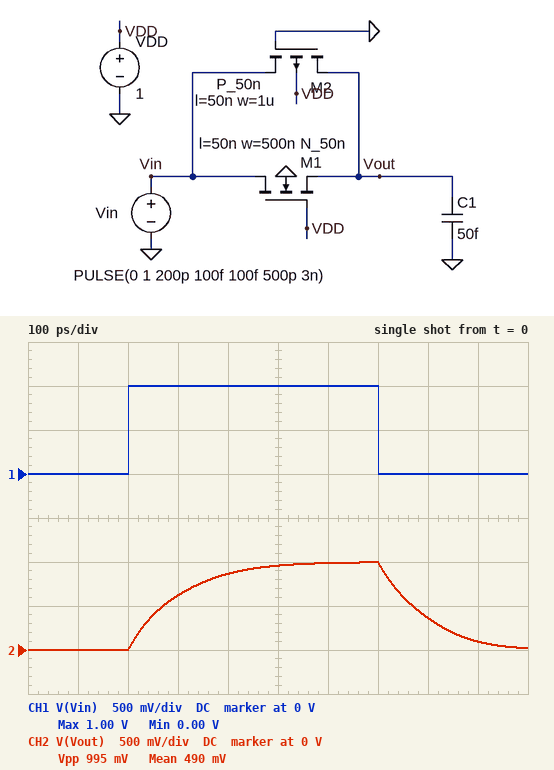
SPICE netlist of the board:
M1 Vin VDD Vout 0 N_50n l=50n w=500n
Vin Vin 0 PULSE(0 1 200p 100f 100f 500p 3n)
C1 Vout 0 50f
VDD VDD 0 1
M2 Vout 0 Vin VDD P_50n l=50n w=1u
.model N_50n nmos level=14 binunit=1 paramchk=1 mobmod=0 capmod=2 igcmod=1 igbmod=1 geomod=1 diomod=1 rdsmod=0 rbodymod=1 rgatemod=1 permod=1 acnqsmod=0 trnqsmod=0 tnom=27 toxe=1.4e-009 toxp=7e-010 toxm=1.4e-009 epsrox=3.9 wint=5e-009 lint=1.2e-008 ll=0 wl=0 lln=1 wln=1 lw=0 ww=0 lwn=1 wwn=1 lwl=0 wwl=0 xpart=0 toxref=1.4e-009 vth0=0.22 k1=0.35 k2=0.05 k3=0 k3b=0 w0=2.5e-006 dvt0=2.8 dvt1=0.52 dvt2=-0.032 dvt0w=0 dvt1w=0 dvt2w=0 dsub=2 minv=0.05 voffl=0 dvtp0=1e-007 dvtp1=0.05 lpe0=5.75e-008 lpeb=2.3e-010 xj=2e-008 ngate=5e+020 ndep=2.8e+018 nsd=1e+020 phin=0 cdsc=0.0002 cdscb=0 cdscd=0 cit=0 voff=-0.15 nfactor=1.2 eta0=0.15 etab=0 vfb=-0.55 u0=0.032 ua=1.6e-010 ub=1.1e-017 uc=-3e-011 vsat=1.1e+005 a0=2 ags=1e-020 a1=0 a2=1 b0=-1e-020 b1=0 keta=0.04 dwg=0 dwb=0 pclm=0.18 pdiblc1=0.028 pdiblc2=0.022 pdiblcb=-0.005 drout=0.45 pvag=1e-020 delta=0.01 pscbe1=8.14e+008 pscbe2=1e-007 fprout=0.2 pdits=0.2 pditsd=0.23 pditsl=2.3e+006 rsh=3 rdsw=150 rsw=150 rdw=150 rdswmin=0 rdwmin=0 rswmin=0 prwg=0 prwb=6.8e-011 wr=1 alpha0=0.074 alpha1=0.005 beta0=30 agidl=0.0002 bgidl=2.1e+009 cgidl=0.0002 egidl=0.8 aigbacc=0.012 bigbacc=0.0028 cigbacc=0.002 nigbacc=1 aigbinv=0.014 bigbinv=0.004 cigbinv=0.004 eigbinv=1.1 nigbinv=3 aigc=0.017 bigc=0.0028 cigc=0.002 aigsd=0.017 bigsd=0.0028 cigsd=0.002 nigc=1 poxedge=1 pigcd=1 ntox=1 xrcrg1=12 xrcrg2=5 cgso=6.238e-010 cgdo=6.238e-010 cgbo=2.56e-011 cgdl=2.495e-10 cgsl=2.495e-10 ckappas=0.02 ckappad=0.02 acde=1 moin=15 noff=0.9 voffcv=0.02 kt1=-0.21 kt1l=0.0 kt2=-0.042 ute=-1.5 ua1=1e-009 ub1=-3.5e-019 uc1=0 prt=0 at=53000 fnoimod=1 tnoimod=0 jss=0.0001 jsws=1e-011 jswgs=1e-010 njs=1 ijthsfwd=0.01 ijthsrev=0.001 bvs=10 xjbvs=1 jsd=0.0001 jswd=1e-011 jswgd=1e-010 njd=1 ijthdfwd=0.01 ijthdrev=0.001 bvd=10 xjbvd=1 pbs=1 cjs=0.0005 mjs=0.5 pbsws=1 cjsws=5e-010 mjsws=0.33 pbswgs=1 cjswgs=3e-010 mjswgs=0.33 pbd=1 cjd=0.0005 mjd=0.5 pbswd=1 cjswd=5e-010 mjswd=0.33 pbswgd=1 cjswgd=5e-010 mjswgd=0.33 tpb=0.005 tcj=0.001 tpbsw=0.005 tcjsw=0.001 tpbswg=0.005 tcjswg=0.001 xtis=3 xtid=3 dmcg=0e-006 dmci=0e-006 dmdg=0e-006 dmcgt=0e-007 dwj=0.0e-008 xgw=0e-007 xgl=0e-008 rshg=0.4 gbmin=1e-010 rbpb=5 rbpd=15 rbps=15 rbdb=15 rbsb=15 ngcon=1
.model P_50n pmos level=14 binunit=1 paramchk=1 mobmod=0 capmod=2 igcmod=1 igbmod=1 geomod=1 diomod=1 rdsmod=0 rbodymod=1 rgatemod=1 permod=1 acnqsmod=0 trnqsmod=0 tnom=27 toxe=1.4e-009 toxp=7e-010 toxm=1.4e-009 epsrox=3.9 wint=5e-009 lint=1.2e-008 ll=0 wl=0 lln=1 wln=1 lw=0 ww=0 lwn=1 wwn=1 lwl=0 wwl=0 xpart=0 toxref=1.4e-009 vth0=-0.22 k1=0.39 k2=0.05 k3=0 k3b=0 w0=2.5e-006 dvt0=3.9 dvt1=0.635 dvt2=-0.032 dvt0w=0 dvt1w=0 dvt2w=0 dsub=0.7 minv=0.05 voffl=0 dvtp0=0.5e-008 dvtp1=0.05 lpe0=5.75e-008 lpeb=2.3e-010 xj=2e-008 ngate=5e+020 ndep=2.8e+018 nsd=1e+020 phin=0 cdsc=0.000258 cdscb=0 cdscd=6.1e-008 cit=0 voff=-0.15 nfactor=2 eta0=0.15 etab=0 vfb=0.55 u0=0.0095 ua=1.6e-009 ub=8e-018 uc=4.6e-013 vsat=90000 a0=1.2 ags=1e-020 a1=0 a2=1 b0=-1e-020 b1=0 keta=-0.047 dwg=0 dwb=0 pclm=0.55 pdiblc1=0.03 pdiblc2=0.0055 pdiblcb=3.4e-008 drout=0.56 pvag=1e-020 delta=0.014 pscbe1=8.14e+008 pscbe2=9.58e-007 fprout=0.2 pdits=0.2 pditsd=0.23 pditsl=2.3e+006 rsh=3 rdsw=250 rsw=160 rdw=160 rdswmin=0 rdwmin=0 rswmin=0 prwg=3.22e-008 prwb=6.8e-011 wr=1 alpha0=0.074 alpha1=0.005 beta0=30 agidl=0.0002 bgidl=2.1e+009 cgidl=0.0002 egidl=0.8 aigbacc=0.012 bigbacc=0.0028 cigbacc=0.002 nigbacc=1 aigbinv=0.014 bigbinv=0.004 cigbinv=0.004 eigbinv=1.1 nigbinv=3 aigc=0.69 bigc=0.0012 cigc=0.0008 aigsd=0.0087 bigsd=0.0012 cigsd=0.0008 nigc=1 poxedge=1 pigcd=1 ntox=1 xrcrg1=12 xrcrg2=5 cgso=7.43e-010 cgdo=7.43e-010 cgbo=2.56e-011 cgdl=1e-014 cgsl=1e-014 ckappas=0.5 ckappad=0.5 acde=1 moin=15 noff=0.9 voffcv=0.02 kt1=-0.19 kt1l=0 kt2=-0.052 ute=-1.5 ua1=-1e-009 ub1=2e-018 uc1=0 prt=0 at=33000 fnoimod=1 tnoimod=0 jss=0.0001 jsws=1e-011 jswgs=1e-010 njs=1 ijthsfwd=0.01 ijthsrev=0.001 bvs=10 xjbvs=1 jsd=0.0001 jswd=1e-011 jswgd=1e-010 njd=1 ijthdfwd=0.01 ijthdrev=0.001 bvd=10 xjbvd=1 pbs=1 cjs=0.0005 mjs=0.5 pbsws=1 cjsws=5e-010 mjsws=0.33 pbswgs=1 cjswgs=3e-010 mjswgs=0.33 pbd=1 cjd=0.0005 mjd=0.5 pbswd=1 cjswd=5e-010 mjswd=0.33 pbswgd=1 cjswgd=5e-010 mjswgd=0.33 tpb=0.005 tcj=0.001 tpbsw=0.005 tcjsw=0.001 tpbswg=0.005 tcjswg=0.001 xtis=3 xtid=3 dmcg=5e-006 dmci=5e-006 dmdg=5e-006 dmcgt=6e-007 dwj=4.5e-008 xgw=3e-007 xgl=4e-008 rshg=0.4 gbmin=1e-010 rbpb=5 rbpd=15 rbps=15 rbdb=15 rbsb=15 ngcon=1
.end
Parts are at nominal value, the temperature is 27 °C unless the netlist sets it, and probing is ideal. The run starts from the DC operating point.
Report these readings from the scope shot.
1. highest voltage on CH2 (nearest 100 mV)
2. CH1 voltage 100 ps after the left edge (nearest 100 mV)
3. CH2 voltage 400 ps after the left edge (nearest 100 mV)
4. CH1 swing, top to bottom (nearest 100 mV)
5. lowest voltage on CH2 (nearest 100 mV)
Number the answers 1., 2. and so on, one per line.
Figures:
1. 1.0 V
2. 0 V
3. 900 mV
4. 1.0 V
5. 0 V
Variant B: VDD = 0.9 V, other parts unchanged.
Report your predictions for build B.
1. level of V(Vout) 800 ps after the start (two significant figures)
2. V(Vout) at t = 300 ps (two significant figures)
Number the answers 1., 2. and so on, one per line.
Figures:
1. 400 mV
2. 590 mV
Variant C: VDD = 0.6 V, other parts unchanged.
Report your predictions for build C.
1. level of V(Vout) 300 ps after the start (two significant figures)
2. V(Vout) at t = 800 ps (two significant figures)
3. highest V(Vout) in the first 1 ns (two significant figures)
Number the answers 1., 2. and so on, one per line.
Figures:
1. 550 mV
2. 540 mV
3. 1.0 V
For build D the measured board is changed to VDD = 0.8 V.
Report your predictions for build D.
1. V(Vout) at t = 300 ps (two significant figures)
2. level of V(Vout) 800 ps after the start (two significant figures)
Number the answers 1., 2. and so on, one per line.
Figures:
1. 570 mV
2. 450 mV
